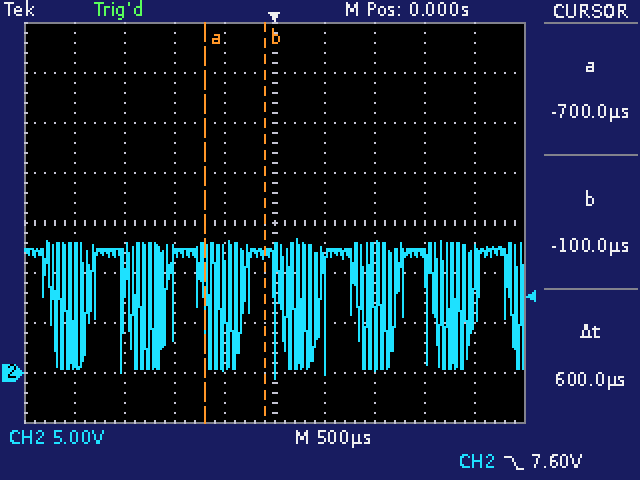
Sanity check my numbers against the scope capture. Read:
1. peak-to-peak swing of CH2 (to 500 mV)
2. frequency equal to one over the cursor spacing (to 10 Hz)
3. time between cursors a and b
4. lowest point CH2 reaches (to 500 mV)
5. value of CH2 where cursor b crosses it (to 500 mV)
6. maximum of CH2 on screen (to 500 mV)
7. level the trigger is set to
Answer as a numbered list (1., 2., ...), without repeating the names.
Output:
1. 14.0 V
2. 1.67 kHz
3. 600 µs
4. -500 mV
5. 12.0 V
6. 13.5 V
7. 7.60 V
